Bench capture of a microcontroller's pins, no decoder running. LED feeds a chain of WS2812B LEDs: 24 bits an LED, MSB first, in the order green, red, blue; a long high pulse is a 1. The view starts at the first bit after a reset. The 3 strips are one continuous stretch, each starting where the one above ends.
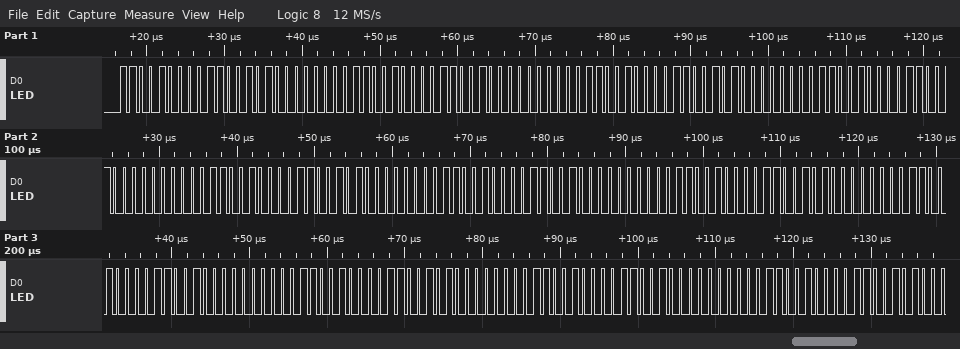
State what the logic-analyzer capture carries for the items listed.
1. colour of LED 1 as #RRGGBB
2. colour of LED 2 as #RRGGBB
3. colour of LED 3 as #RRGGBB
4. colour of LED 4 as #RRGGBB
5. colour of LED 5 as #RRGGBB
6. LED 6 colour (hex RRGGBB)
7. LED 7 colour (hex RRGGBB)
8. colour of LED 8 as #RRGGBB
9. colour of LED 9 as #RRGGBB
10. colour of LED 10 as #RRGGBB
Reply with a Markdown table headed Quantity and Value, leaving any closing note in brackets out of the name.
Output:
| Quantity | Value |
|---|---|
| colour of LED 1 as #RRGGBB | #65C800 |
| colour of LED 2 as #RRGGBB | #64C800 |
| colour of LED 3 as #RRGGBB | #65C800 |
| colour of LED 4 as #RRGGBB | #64C800 |
| colour of LED 5 as #RRGGBB | #65C800 |
| LED 6 colour | #64C800 |
| LED 7 colour | #65C800 |
| colour of LED 8 as #RRGGBB | #64C800 |
| colour of LED 9 as #RRGGBB | #65C800 |
| colour of LED 10 as #RRGGBB | #64C800 |
